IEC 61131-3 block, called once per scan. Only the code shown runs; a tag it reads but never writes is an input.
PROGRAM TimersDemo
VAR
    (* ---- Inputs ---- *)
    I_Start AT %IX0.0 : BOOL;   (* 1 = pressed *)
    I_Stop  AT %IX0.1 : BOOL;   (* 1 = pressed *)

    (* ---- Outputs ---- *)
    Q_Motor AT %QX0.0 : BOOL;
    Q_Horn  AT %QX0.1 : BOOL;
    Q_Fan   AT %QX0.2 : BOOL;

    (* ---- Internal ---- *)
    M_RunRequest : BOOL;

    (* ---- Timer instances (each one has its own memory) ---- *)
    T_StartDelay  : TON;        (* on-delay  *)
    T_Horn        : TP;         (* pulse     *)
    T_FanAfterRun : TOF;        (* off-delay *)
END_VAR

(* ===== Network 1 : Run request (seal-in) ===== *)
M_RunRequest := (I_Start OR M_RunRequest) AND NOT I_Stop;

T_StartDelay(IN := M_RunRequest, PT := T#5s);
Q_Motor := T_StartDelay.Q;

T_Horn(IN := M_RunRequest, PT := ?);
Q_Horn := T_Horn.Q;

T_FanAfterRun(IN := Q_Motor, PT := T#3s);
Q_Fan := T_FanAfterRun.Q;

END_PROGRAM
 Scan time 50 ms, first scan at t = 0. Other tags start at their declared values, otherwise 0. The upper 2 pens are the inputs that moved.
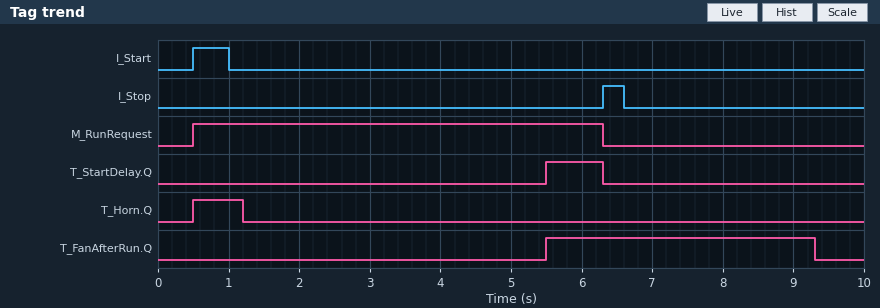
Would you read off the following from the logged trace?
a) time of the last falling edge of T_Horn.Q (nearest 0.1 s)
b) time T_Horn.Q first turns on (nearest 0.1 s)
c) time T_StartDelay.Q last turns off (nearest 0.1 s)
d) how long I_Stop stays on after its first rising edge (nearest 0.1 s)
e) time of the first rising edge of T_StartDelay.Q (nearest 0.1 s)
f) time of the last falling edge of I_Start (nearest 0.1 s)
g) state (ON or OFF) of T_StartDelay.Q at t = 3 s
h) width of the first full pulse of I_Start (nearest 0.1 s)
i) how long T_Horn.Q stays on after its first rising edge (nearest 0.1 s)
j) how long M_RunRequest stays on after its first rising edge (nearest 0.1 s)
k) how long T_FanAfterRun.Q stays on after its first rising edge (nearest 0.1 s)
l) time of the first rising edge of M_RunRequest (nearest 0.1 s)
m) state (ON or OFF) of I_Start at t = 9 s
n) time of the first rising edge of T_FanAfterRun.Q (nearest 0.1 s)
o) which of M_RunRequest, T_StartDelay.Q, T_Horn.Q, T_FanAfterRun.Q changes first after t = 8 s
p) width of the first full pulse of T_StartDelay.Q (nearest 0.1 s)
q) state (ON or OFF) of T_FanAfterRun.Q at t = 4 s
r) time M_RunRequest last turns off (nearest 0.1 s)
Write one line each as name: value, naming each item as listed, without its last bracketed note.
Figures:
time of the last falling edge of T_Horn.Q: 1.2 s
time T_Horn.Q first turns on: 0.5 s
time T_StartDelay.Q last turns off: 6.3 s
how long I_Stop stays on after its first rising edge: 0.3 s
time of the first rising edge of T_StartDelay.Q: 5.5 s
time of the last falling edge of I_Start: 1.0 s
state (ON or OFF) of T_StartDelay.Q at t = 3 s: OFF
width of the first full pulse of I_Start: 0.5 s
how long T_Horn.Q stays on after its first rising edge: 0.7 s
how long M_RunRequest stays on after its first rising edge: 5.8 s
how long T_FanAfterRun.Q stays on after its first rising edge: 3.8 s
time of the first rising edge of M_RunRequest: 0.5 s
state (ON or OFF) of I_Start at t = 9 s: OFF
time of the first rising edge of T_FanAfterRun.Q: 5.5 s
which of M_RunRequest, T_StartDelay.Q, T_Horn.Q, T_FanAfterRun.Q changes first after t = 8 s: T_FanAfterRun.Q
width of the first full pulse of T_StartDelay.Q: 0.8 s
state (ON or OFF) of T_FanAfterRun.Q at t = 4 s: OFF
time M_RunRequest last turns off: 6.3 s
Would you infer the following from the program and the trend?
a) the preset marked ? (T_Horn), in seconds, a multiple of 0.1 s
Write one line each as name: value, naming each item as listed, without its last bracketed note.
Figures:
the preset marked ? (T_Horn), in seconds, a multiple of 0.1 s: 0.7 s
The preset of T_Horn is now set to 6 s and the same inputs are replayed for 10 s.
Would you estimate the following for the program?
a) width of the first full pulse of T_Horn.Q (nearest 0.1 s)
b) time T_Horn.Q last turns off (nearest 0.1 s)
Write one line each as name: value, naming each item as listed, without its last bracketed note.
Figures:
width of the first full pulse of T_Horn.Q: 6.0 s
time T_Horn.Q last turns off: 6.5 s
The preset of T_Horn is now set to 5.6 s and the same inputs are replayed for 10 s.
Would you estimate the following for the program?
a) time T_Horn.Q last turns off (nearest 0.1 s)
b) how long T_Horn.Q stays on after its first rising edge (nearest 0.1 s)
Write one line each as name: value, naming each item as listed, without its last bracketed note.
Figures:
time T_Horn.Q last turns off: 6.1 s
how long T_Horn.Q stays on after its first rising edge: 5.6 s
